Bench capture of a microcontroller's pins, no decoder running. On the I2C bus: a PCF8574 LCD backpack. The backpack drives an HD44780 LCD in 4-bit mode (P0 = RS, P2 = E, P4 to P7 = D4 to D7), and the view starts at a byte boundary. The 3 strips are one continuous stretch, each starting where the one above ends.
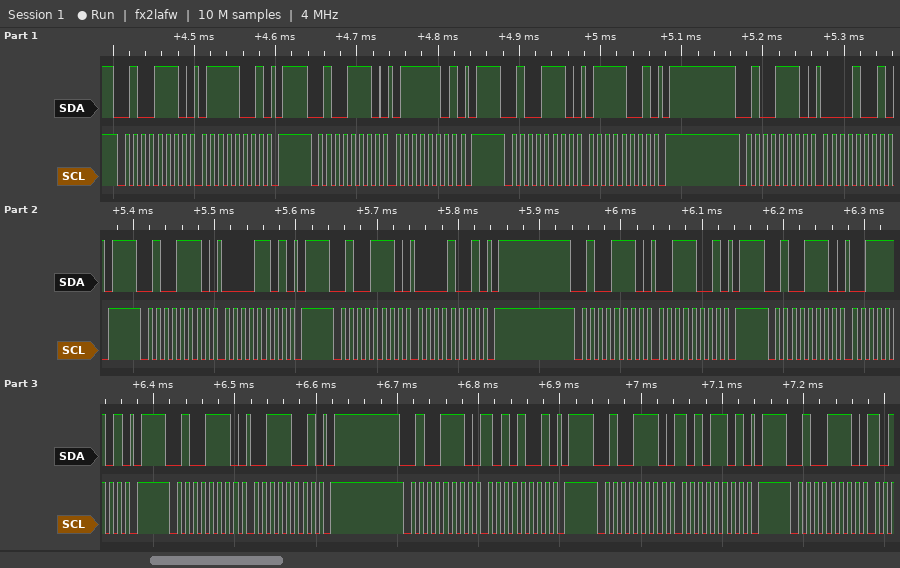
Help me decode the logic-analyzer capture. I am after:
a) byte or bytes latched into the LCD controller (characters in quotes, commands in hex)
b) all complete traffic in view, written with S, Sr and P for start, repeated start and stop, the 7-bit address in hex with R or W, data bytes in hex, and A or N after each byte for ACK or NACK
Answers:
'p'
S 27W A 79 A P S 27W A 7D A P S 27W A 79 A P S 27W A 09 A P S 27W A 0D A P S 27W A 09 A P S 27W A 39 A P S 27W A 3D A P S 27W A 39 A P S 27W A A9 A P S 27W A AD A P S 27W A
